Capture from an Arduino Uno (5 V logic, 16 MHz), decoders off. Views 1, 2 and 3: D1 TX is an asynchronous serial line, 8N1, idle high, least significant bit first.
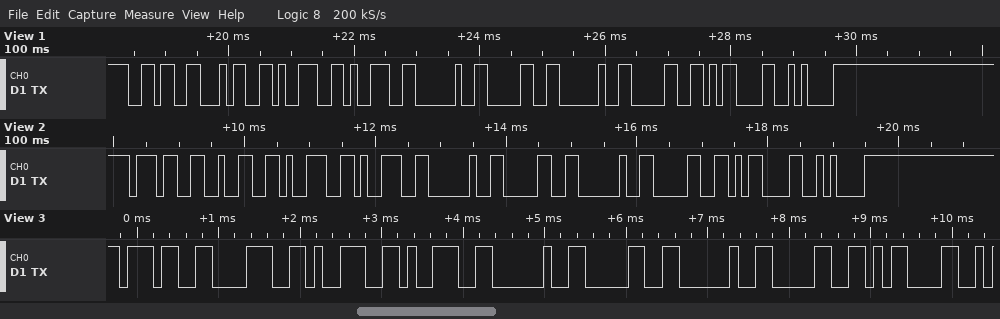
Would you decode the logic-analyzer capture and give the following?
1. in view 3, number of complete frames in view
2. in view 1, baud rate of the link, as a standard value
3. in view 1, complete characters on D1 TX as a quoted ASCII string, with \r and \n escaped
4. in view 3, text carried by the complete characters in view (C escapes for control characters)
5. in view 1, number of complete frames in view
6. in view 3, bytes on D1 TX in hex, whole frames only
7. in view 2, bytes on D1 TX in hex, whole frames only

9
9600 baud
"6499 0 0\r\n"
"7899 0 0\r"
10
37 38 39 39 20 30 20 30 0D
37 32 39 39 20 30 20 30 0D 0A
